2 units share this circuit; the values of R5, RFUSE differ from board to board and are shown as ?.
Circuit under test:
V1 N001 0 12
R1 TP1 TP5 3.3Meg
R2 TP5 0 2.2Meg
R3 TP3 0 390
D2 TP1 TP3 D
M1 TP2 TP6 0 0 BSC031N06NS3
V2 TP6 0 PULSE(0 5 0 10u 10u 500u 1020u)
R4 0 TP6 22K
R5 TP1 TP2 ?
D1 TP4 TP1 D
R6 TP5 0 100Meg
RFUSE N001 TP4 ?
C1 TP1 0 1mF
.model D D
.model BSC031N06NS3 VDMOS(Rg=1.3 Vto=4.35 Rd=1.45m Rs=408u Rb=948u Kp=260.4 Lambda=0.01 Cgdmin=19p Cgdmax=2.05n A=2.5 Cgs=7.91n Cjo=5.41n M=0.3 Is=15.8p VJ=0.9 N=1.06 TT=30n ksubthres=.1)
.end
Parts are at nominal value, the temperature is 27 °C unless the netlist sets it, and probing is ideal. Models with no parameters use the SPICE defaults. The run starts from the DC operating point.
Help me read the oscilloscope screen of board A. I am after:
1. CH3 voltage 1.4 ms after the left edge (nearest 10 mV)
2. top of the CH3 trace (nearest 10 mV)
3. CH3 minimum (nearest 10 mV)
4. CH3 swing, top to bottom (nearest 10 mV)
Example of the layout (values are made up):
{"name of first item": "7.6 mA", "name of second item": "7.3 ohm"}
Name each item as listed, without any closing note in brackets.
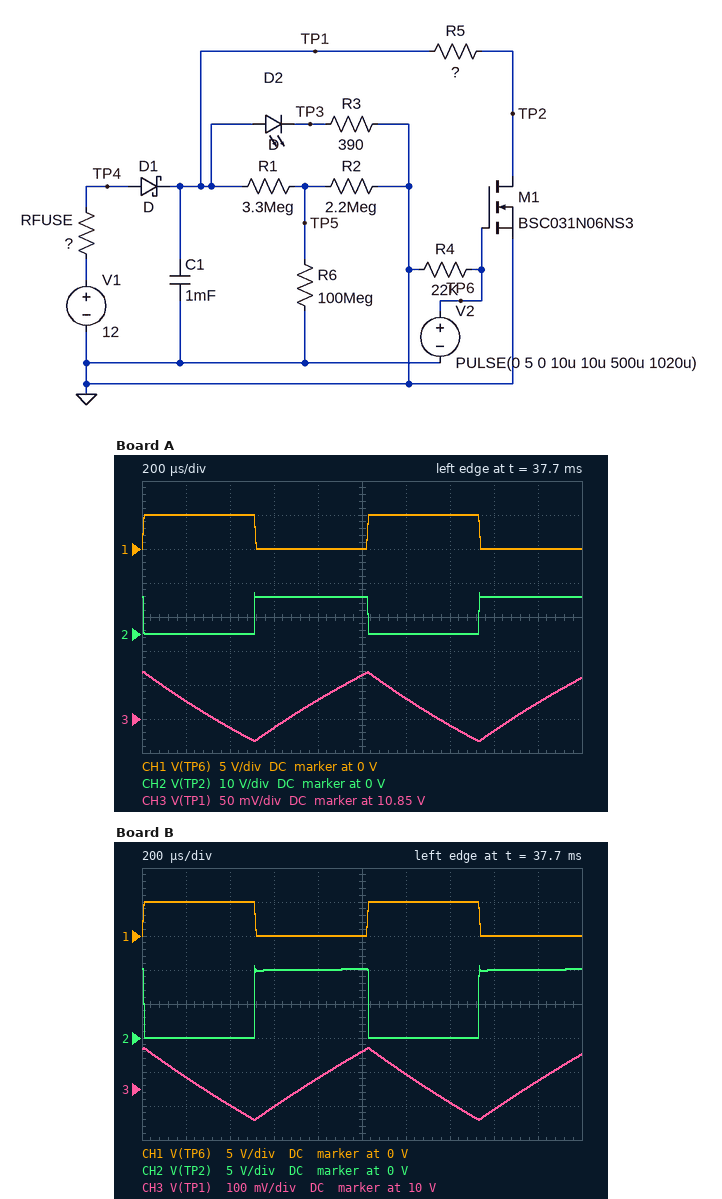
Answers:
{"CH3 voltage 1.4 ms after the left edge": "10.84 V", "top of the CH3 trace": "10.92 V", "CH3 minimum": "10.82 V", "CH3 swing, top to bottom": "100 mV"}
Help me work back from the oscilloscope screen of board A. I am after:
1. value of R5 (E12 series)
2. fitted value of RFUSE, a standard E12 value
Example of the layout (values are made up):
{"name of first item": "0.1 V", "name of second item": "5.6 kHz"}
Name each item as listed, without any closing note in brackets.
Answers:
{"value of R5": "27 Ω", "fitted value of RFUSE, a standard E12 value": "1.5 Ω"}
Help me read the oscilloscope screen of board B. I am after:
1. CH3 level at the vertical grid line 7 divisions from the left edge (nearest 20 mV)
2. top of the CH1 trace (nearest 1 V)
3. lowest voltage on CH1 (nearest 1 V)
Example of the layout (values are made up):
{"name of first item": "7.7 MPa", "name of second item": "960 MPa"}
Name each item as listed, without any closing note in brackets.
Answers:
{"CH3 level at the vertical grid line 7 divisions from the left edge": "9.96 V", "top of the CH1 trace": "5 V", "lowest voltage on CH1": "0 V"}
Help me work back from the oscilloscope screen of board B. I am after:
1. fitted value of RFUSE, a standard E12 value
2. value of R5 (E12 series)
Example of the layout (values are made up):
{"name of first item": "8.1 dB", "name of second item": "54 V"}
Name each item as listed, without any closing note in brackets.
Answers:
{"fitted value of RFUSE, a standard E12 value": "2.7 Ω", "value of R5": "12 Ω"}
